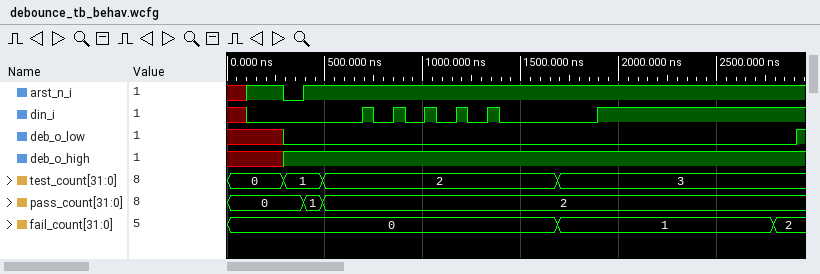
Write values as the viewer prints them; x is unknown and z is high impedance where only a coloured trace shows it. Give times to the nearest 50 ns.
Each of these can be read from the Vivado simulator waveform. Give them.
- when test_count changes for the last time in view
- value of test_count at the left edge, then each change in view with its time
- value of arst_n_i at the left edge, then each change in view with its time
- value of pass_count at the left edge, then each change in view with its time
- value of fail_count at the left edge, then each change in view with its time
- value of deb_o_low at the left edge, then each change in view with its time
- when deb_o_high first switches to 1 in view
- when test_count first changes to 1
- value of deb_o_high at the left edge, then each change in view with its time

1700 ns
0, 1 at 300 ns, 2 at 500 ns, 3 at 1700 ns
x, 1 at 100 ns, 0 at 300 ns, 1 at 400 ns
0, 1 at 400 ns, 2 at 500 ns
0, 1 at 1700 ns, 2 at 2800 ns
x, 0 at 300 ns, 1 at 2900 ns
300 ns
300 ns
x, 1 at 300 ns
